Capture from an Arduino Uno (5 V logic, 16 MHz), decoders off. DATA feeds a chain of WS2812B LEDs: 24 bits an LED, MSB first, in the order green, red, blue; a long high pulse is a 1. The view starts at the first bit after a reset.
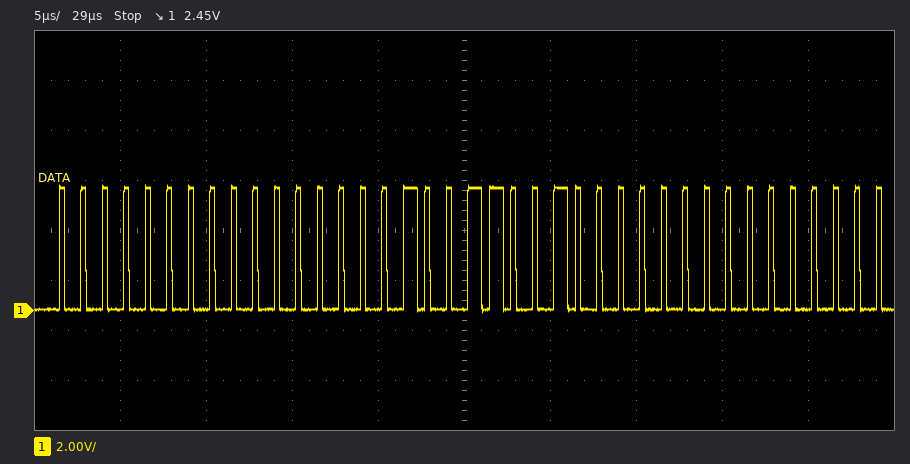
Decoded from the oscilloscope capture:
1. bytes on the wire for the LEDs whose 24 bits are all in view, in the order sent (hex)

00 00 99
